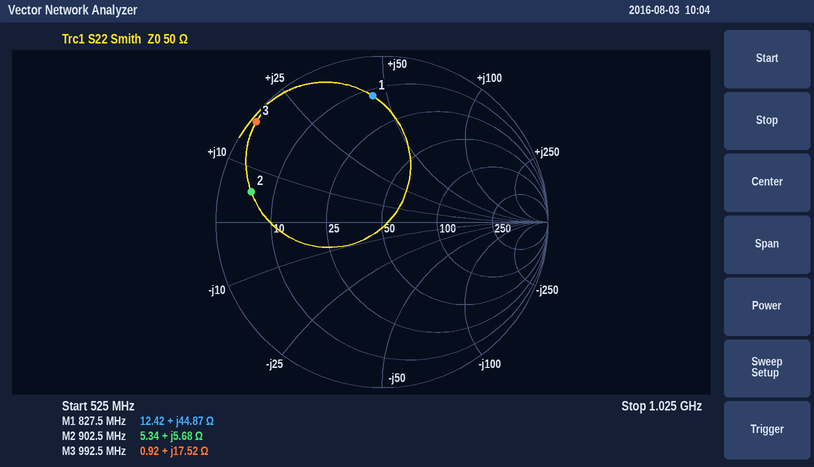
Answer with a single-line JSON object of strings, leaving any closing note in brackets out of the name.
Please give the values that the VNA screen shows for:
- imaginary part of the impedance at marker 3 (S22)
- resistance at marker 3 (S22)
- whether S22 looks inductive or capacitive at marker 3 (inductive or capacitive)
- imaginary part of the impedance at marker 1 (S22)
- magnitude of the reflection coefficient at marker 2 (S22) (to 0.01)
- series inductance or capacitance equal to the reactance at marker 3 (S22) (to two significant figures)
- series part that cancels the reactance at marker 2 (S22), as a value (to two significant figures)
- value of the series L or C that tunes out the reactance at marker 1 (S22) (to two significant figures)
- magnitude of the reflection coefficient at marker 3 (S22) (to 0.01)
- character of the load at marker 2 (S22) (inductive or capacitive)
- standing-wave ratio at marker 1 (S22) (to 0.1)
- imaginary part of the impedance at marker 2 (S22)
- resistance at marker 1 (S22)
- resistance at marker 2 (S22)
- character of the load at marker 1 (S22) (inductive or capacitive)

{"imaginary part of the impedance at marker 3": "+17.52 Ω", "resistance at marker 3": "0.92 Ω", "whether S22 looks inductive or capacitive at marker 3": "inductive", "imaginary part of the impedance at marker 1": "+44.87 Ω", "magnitude of the reflection coefficient at marker 2 (S22)": "0.81", "series inductance or capacitance equal to the reactance at marker 3 (S22)": "2.8 nH", "series part that cancels the reactance at marker 2 (S22), as a value": "31 pF", "value of the series L or C that tunes out the reactance at marker 1 (S22)": "4.3 pF", "magnitude of the reflection coefficient at marker 3 (S22)": "0.97", "character of the load at marker 2 (S22)": "inductive", "standing-wave ratio at marker 1 (S22)": "7.4", "imaginary part of the impedance at marker 2": "+5.68 Ω", "resistance at marker 1": "12.42 Ω", "resistance at marker 2": "5.34 Ω", "character of the load at marker 1 (S22)": "inductive"}
